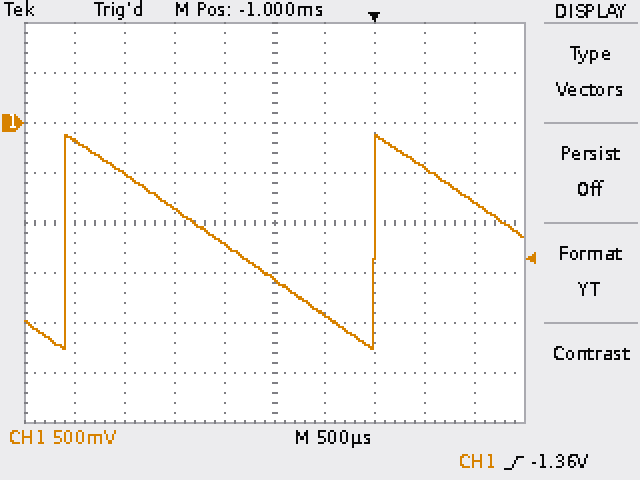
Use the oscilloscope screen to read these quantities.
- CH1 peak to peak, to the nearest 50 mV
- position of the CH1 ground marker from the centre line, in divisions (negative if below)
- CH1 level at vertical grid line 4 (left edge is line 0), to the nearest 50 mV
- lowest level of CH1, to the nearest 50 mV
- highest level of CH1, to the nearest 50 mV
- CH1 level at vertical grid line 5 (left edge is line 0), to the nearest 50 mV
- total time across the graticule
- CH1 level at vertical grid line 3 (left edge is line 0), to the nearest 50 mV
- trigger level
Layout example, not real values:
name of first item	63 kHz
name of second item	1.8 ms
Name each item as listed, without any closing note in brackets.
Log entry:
CH1 peak to peak, to the nearest 50 mV	2.15 V
position of the CH1 ground marker from the centre line, in divisions	+2.0 div
CH1 level at vertical grid line 4 (left edge is line 0), to the nearest 50 mV	-1.20 V
lowest level of CH1, to the nearest 50 mV	-2.25 V
highest level of CH1, to the nearest 50 mV	-100 mV
CH1 level at vertical grid line 5 (left edge is line 0), to the nearest 50 mV	-1.55 V
total time across the graticule	5 ms
CH1 level at vertical grid line 3 (left edge is line 0), to the nearest 50 mV	-850 mV
trigger level	-1.36 V
